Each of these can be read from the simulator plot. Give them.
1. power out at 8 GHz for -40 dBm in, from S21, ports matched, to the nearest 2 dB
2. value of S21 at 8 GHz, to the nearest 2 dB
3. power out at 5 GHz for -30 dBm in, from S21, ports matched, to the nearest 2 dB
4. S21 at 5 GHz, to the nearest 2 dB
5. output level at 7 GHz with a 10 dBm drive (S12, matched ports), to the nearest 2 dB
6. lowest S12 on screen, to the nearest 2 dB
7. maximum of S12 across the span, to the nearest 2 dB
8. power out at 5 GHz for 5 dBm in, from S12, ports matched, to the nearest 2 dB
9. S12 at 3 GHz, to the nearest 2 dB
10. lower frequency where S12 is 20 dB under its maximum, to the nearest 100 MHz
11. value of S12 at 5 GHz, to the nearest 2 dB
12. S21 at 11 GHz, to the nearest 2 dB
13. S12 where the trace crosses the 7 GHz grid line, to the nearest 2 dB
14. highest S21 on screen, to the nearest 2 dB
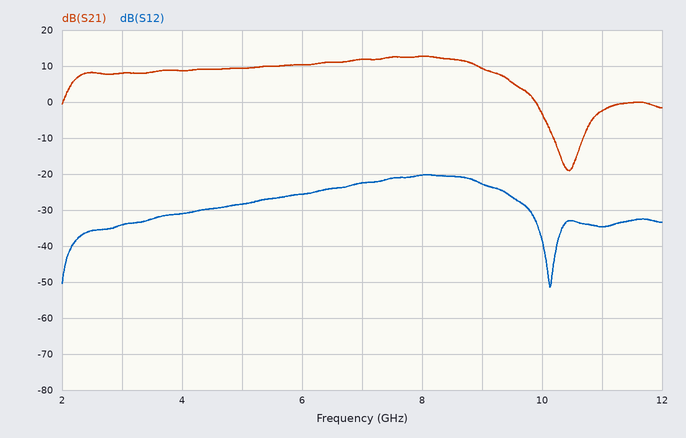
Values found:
-28 dBm
12 dB
-20 dBm
10 dB
-12 dBm
-52 dB
-20 dB
-24 dBm
-34 dB
2.2 GHz
-28 dB
-2 dB
-22 dB
12 dB
